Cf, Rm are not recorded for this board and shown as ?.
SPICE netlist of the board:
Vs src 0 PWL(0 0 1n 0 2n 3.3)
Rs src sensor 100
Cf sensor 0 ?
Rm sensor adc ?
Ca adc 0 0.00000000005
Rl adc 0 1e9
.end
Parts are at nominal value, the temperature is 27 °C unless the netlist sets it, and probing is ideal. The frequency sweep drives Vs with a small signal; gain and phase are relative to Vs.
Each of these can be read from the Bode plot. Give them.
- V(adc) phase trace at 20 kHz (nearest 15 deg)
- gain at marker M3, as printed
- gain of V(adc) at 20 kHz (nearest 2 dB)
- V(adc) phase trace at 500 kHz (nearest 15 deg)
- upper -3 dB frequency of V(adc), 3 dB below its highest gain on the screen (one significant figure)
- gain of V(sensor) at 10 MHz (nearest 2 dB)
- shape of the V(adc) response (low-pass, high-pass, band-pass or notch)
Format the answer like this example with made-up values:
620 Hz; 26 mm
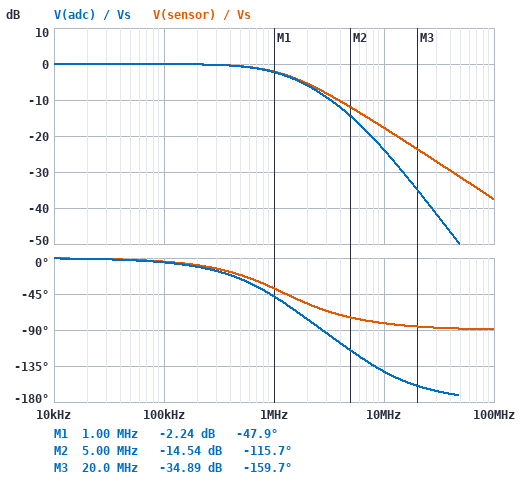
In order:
0 deg; -34.89 dB; 0 dB; -30 deg; 1 MHz; -18 dB; low-pass
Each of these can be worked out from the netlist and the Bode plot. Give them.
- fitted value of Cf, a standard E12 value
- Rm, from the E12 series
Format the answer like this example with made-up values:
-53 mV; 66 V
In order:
1.2 nF; 560 Ω
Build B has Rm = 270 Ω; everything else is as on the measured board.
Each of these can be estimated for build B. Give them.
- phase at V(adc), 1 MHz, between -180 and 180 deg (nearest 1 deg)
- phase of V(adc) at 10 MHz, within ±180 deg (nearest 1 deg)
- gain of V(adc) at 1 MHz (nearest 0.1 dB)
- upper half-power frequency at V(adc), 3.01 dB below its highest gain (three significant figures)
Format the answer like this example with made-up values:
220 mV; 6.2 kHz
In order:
-43 deg; -122 deg; -2.1 dB; 1.25 MHz
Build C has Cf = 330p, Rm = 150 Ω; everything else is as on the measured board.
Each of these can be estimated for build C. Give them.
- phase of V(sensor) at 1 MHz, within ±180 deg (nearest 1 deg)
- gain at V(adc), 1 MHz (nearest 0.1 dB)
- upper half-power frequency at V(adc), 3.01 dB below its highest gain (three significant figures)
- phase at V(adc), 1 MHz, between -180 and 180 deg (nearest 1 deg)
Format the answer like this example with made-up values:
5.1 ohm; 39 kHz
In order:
-13 deg; -0.3 dB; 3.96 MHz; -16 deg
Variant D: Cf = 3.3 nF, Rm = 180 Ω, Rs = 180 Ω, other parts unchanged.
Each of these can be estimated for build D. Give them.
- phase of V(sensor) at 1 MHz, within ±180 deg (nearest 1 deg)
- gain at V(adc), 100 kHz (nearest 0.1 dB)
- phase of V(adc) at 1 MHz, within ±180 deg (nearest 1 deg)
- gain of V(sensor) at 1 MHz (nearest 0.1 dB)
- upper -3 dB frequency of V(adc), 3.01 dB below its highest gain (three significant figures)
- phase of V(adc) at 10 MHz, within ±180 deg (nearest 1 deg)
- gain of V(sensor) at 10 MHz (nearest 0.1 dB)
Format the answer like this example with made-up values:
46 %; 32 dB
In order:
-75 deg; -0.6 dB; -78 deg; -11.9 dB; 264 kHz; -118 deg; -31.5 dB
